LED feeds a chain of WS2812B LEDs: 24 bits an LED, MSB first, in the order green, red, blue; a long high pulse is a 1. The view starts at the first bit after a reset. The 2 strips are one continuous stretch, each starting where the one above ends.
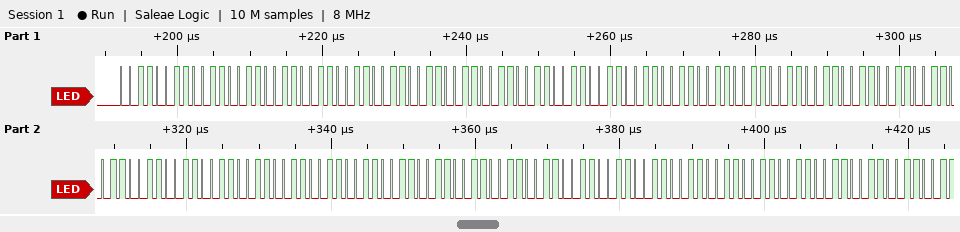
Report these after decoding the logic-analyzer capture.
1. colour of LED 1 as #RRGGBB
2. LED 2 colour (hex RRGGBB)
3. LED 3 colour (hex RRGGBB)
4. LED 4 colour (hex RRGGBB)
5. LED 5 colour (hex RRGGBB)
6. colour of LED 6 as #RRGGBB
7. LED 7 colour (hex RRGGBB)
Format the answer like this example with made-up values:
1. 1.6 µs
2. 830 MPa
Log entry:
1. #333333
2. #333333
3. #333333
4. #333333
5. #333333
6. #333333
7. #333333
